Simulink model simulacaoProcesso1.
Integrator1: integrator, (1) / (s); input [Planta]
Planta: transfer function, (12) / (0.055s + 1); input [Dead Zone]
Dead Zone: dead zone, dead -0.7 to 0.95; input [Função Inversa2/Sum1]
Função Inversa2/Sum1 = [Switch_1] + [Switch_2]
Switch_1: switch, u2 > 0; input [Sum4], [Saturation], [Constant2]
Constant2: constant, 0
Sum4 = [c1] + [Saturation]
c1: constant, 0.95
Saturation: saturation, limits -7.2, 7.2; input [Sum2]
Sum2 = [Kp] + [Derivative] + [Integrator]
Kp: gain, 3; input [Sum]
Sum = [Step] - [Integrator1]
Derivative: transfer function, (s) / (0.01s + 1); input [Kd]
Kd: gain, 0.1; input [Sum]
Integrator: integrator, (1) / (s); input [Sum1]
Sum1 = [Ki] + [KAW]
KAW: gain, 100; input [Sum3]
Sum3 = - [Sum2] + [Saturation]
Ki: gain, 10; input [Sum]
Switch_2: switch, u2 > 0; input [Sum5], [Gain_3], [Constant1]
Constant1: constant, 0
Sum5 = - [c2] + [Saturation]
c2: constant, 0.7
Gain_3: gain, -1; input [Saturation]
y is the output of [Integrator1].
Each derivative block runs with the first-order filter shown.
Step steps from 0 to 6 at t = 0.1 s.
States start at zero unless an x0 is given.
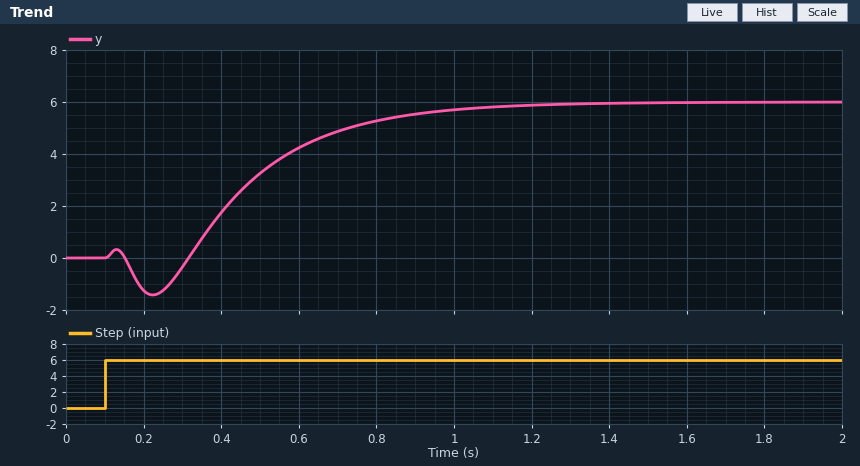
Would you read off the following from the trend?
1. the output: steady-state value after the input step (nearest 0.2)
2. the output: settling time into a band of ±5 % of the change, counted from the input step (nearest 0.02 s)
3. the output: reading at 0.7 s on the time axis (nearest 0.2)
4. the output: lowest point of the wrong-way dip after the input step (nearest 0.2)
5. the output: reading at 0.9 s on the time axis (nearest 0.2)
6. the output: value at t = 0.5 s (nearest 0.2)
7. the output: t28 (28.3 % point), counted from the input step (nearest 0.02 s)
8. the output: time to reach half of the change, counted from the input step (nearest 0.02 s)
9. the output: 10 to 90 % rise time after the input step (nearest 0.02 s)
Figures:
6.0
0.90 s
4.8
-1.4
5.6
3.2
0.30 s
0.38 s
0.50 s
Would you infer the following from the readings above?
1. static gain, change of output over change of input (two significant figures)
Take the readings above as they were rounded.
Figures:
1.0
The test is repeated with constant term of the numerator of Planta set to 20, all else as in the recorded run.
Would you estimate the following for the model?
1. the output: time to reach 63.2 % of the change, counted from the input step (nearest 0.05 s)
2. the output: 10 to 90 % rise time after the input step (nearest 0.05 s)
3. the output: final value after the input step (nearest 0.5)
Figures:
0.45 s
0.55 s
6.0
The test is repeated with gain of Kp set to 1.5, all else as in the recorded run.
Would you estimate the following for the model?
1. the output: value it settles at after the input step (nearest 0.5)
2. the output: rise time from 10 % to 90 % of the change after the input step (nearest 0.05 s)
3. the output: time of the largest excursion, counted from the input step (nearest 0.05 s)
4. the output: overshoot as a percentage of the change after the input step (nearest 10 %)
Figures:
6.0
0.15 s
0.60 s
20 %
